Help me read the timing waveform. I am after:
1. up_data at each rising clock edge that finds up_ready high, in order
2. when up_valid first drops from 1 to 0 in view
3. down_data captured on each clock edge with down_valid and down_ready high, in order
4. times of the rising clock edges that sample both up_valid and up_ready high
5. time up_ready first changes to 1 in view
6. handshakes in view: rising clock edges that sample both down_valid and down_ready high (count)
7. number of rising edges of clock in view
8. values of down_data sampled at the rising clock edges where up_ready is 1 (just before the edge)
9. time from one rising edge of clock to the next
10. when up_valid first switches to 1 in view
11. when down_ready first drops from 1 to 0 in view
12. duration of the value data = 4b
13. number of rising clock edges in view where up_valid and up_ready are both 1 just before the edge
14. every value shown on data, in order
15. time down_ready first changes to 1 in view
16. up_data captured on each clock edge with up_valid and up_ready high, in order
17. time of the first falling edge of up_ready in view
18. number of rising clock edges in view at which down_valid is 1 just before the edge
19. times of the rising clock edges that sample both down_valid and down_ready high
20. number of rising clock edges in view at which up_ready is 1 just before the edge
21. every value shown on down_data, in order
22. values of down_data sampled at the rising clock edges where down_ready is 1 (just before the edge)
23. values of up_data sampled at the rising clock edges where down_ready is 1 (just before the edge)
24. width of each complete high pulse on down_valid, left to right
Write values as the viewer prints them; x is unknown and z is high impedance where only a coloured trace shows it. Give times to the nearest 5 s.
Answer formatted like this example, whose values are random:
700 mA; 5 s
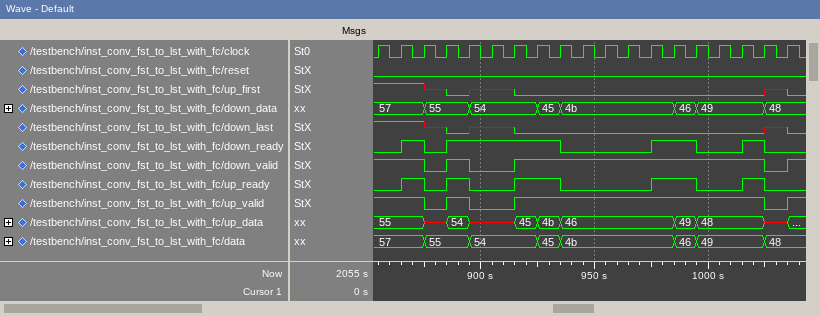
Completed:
55, 54, 45, 4b, 46, 49, 48; 875 s; 57, 55, 54, 45, 4b, 46, 49; 875 s, 895 s, 925 s, 935 s, 985 s, 995 s, 1025 s; 865 s; 7; 19; 57, 55, 54, 45, 4b, 46, 49; 10 s; 885 s; 875 s; 50 s; 7; 57, 55, 54, 45, 4b, 46, 49, 48; 865 s; 55, 54, 45, 4b, 46, 49, 48; 875 s; 15; 875 s, 895 s, 925 s, 935 s, 985 s, 995 s, 1025 s; 7; 57, 55, 54, 45, 4b, 46, 49, 48; 57, 55, 54, 54, 54, 45, 4b, 46, 49; 55, 54, x, x, 45, 4b, 46, 49, 48; 10 s, 110 s
